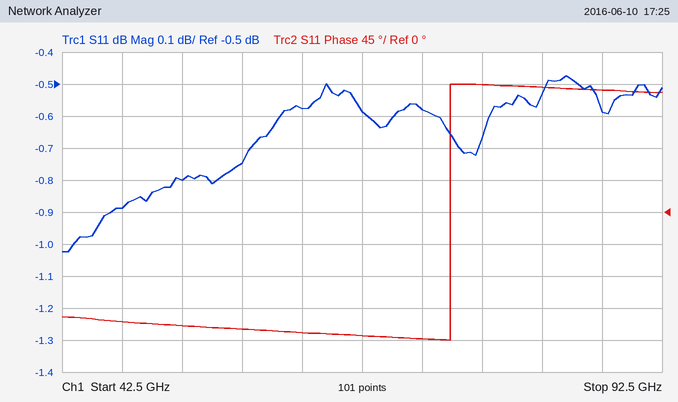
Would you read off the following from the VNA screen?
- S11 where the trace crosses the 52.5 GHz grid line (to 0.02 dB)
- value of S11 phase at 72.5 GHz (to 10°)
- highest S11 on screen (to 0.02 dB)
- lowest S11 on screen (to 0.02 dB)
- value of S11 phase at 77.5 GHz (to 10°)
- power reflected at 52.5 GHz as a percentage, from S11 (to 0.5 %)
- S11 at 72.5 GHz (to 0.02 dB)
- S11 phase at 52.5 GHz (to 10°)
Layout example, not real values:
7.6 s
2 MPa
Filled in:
-0.80 dB
-180°
-0.48 dB
-1.02 dB
180°
83.0 %
-0.58 dB
-160°
